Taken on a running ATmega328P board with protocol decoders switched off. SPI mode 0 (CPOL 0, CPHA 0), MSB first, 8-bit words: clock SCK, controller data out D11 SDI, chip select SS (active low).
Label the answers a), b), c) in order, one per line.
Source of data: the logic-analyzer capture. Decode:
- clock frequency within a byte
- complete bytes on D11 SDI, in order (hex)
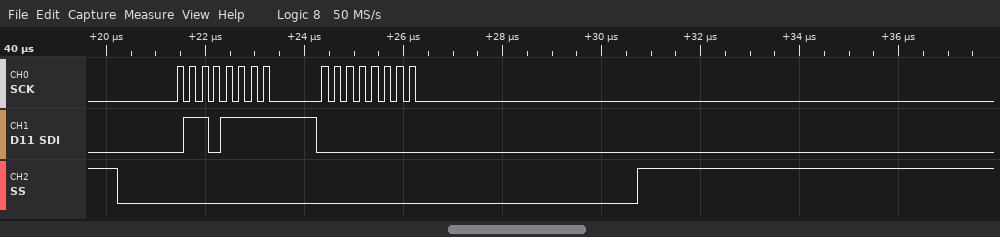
a) 4 MHz
b) 0x6F 0x00
